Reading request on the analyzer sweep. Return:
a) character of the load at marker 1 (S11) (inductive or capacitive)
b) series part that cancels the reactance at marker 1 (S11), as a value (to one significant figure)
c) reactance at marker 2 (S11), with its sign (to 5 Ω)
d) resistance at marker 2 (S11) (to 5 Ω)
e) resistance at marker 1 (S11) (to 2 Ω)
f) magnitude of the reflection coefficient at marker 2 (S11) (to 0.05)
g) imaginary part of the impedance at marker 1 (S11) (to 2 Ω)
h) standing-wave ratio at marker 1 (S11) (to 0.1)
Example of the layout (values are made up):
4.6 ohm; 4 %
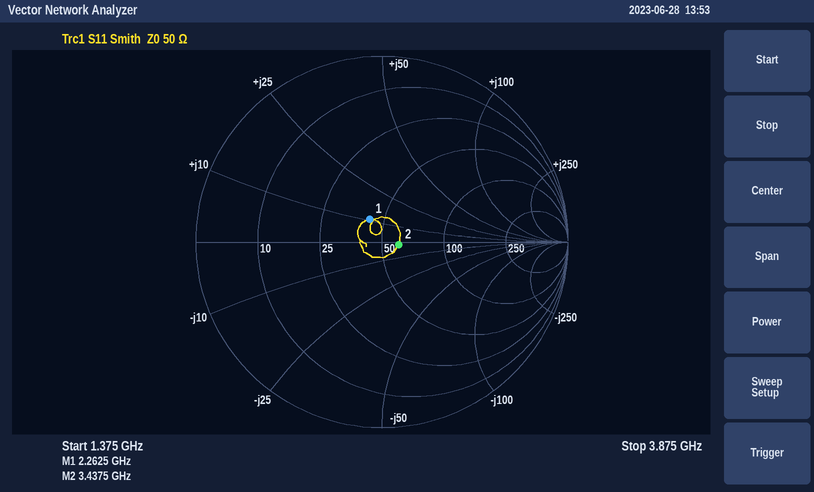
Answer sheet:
inductive; 7 pF; 0 Ω; 60 Ω; 42 Ω; 0.10; +10 Ω; 1.3
